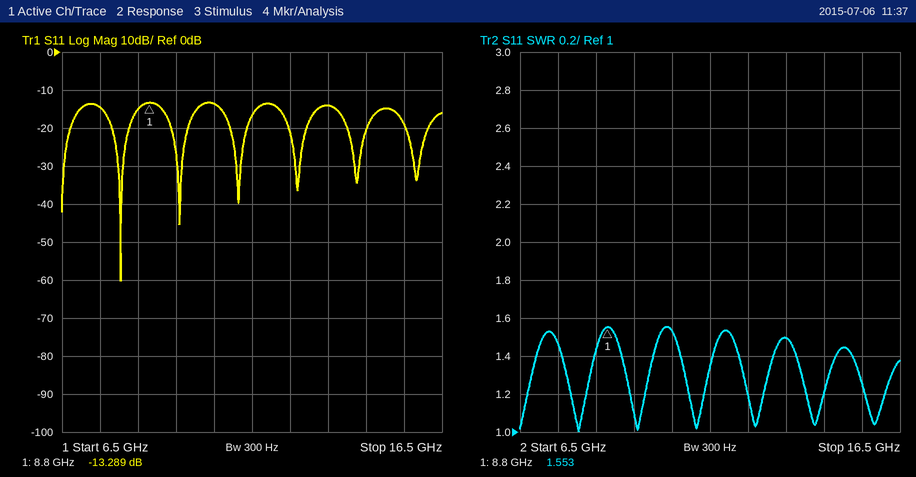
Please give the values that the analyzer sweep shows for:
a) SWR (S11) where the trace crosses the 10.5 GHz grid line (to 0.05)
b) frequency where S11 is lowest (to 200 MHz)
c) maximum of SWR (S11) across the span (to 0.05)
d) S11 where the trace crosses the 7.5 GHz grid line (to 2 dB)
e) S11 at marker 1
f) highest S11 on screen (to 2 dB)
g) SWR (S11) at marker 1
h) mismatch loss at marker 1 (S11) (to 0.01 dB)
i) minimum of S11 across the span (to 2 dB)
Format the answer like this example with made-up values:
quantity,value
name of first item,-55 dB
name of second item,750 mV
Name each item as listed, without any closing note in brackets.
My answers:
quantity,value
SWR (S11) where the trace crosses the 10.5 GHz grid line,1.55
frequency where S11 is lowest,8.0 GHz
maximum of SWR (S11) across the span,1.55
S11 where the trace crosses the 7.5 GHz grid line,-14 dB
S11 at marker 1,-13.289 dB
highest S11 on screen,-14 dB
SWR (S11) at marker 1,1.553
mismatch loss at marker 1 (S11),0.21 dB
minimum of S11 across the span,-60 dB
